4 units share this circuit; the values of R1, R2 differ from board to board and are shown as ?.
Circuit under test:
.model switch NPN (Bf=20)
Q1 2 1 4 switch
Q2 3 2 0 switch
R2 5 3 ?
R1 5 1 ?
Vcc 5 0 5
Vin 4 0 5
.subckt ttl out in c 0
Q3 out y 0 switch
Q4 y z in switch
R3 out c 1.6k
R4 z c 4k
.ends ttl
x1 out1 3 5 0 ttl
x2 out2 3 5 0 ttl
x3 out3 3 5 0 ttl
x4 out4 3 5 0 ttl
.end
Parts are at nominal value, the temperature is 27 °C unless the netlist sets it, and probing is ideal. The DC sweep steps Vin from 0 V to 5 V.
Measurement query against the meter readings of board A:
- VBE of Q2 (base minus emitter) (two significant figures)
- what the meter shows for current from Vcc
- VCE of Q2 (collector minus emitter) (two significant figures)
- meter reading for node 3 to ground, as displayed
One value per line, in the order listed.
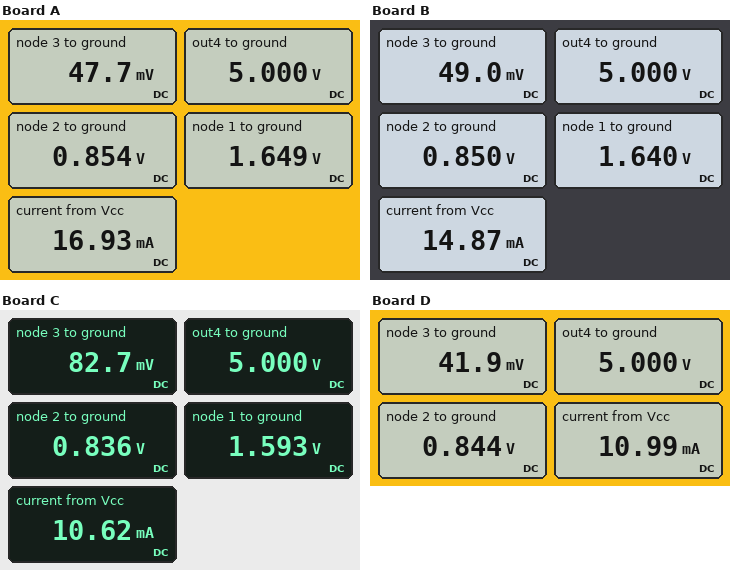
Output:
850 mV
16.93 mA
48 mV
47.7 mV
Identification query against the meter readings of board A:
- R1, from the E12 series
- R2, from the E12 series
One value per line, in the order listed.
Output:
1.5 kΩ
470 Ω
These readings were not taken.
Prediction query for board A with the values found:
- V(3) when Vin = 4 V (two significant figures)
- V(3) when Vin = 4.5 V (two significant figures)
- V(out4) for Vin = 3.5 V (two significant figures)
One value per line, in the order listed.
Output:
48 mV
48 mV
5.0 V
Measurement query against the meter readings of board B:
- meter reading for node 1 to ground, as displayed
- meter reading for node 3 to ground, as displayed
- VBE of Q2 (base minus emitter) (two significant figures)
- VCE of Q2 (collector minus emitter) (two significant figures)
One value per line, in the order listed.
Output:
1.640 V
49.0 mV
850 mV
49 mV
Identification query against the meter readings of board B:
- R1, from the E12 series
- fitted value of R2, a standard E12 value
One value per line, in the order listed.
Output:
1.8 kΩ
560 Ω
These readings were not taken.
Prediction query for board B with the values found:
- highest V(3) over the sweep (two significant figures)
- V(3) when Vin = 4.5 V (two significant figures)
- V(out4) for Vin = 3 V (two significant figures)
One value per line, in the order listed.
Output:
3.1 V
49 mV
5.0 V
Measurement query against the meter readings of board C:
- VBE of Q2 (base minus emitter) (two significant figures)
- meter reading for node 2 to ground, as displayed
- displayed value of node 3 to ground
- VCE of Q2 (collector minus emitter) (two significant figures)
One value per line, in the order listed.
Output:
840 mV
0.836 V
82.7 mV
83 mV
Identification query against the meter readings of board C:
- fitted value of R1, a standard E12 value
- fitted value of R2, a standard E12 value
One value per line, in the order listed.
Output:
6.8 kΩ
820 Ω
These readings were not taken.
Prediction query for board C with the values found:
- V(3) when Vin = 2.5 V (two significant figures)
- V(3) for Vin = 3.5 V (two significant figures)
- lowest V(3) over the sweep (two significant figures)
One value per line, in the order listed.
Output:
83 mV
83 mV
83 mV
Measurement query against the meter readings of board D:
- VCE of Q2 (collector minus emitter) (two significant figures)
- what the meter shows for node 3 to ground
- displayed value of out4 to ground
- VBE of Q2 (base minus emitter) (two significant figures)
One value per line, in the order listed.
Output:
42 mV
41.9 mV
5.000 V
840 mV
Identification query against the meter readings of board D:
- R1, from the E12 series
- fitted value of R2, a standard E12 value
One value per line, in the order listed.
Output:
1.8 kΩ
1 kΩ
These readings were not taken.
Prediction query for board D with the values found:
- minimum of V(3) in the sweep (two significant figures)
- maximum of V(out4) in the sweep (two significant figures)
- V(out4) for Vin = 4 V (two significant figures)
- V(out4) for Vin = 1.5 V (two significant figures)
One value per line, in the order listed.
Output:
42 mV
5.0 V
5.0 V
5.0 V
